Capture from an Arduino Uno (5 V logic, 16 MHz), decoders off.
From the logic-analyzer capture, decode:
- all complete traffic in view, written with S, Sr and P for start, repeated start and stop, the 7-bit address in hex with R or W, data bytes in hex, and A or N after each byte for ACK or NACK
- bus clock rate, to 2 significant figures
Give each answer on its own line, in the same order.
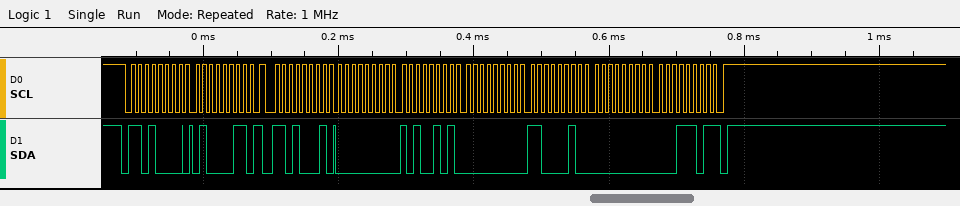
S 68W A 43 A Sr 68R A 00 A A5 A 00 A C2 A 00 A 1D N P
100 kHz
